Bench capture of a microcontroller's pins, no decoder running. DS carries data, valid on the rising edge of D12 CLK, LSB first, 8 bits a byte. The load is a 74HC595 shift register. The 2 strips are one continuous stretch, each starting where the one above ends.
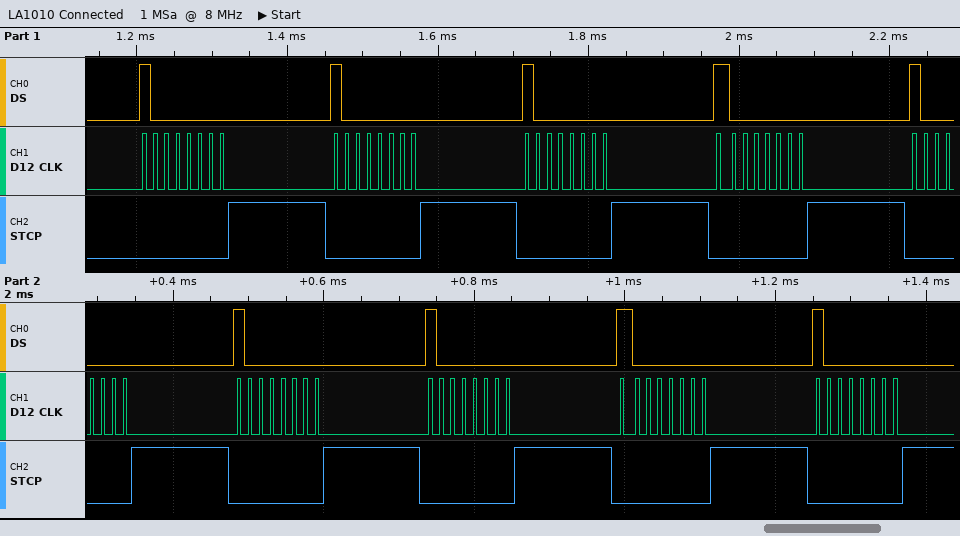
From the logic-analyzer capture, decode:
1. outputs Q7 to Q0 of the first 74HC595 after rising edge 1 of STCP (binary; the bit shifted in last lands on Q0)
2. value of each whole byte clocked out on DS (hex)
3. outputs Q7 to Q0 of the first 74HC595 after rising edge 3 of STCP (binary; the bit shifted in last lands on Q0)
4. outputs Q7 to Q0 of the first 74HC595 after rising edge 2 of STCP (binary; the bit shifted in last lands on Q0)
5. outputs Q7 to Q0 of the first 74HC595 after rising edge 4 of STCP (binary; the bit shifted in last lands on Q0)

10000000
01 01 01 01 01 01 01 01 01
10000000
10000000
10000000
